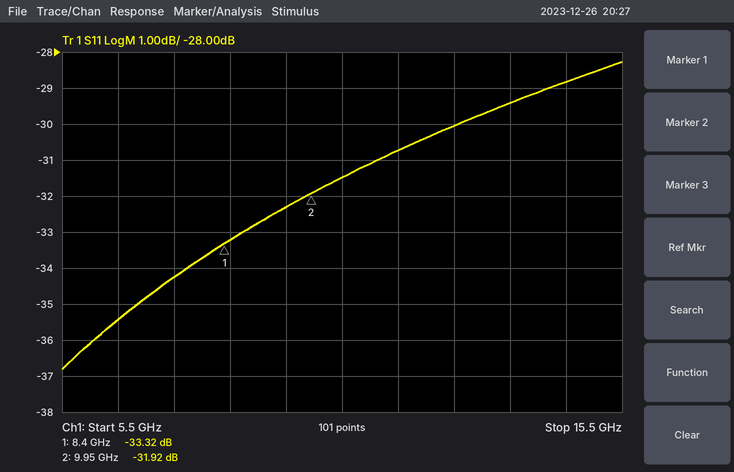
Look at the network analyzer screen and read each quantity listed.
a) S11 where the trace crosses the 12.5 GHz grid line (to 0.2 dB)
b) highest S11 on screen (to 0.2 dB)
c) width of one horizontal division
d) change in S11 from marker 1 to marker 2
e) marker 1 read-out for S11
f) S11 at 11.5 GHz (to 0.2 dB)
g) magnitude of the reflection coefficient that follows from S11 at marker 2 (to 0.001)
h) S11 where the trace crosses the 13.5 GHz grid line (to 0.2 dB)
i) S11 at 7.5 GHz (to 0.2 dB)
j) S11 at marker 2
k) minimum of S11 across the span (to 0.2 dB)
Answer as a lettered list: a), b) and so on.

a) -30.0 dB
b) -28.2 dB
c) 1 GHz
d) 1.40 dB
e) -33.32 dB
f) -30.8 dB
g) 0.025
h) -29.4 dB
i) -34.2 dB
j) -31.92 dB
k) -36.8 dB
